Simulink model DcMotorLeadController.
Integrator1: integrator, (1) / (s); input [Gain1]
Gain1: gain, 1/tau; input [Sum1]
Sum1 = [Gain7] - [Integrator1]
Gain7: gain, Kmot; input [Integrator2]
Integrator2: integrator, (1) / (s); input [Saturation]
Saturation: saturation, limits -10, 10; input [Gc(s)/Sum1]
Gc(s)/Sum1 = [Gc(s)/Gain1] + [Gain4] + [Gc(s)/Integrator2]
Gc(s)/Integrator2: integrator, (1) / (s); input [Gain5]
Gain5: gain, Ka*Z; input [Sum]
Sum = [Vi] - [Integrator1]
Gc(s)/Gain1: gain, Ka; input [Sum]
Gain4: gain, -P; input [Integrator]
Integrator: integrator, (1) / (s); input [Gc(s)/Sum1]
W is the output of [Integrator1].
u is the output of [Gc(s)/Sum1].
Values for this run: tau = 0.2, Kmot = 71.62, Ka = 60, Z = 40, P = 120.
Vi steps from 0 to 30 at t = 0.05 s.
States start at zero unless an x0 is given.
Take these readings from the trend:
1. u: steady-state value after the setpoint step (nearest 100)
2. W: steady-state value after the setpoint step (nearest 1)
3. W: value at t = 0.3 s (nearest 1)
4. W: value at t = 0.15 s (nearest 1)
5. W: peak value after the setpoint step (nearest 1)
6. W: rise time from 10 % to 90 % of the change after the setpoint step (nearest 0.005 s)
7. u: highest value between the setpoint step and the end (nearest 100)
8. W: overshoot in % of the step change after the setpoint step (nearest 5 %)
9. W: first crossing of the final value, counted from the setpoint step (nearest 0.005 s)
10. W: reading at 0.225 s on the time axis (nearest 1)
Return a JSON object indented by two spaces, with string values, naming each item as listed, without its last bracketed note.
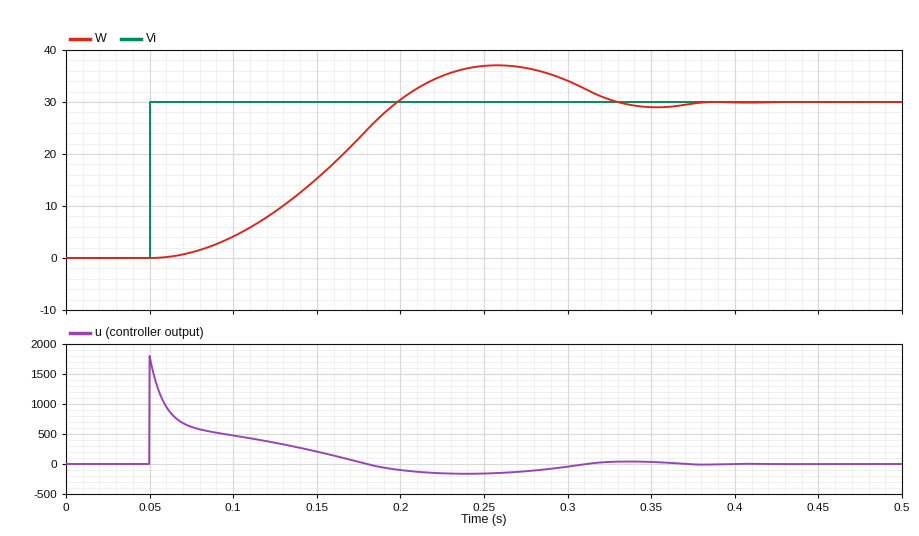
{
  "u: steady-state value after the setpoint step": "0",
  "W: steady-state value after the setpoint step": "30",
  "W: value at t = 0.3 s": "34",
  "W: value at t = 0.15 s": "15",
  "W: peak value after the setpoint step": "37",
  "W: rise time from 10 % to 90 % of the change after the setpoint step": "0.095 s",
  "u: highest value between the setpoint step and the end": "1800",
  "W: overshoot in % of the step change after the setpoint step": "25 %",
  "W: first crossing of the final value, counted from the setpoint step": "0.150 s",
  "W: reading at 0.225 s on the time axis": "35"
}
